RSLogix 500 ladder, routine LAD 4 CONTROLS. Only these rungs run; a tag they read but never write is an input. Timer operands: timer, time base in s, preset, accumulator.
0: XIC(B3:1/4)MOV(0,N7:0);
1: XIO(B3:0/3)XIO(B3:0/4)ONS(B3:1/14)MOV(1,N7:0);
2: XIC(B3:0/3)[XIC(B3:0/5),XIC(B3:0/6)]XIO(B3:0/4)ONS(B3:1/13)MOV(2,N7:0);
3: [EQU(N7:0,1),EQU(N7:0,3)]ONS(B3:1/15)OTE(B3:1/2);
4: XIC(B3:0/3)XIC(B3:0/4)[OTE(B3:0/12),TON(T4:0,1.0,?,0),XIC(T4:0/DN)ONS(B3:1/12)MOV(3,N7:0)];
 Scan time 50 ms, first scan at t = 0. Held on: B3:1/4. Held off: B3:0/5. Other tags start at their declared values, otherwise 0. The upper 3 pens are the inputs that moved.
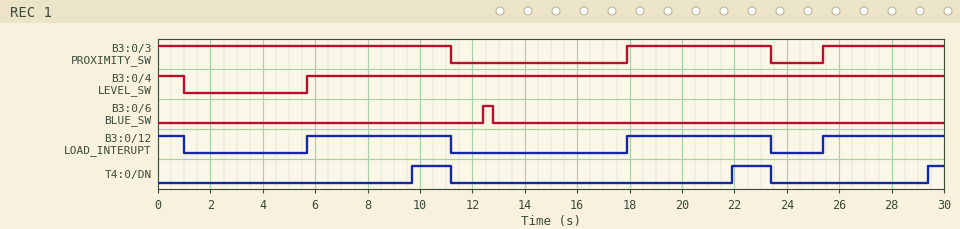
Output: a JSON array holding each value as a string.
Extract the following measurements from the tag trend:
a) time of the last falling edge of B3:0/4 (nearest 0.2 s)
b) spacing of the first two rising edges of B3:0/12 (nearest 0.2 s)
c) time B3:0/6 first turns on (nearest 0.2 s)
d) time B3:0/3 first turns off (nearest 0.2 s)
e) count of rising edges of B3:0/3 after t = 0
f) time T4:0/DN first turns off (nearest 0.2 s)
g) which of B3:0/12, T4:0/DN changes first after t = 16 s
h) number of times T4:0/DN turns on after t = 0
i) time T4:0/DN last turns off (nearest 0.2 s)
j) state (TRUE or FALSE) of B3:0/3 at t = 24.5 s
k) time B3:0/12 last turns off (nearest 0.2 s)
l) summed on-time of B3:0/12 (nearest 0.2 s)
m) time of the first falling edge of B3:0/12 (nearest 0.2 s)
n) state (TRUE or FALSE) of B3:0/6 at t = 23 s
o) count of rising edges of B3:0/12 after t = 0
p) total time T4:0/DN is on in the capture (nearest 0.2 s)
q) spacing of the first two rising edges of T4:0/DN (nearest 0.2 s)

["1.0 s", "12.2 s", "12.4 s", "11.2 s", "2", "11.2 s", "B3:0/12", "3", "23.4 s", "FALSE", "23.4 s", "16.6 s", "1.0 s", "FALSE", "3", "3.6 s", "12.2 s"]
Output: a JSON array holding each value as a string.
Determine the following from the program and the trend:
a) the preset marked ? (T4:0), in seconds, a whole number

["4 s"]
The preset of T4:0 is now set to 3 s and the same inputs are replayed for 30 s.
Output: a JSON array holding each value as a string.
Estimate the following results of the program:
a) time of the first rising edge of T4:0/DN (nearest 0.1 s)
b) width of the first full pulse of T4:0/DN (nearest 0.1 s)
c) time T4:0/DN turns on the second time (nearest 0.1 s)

["8.7 s", "2.5 s", "20.9 s"]
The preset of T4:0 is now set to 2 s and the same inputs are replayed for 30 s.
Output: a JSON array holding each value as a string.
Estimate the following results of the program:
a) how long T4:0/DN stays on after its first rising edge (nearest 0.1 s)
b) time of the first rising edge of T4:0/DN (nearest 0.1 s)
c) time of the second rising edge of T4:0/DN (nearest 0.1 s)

["3.5 s", "7.7 s", "19.9 s"]
